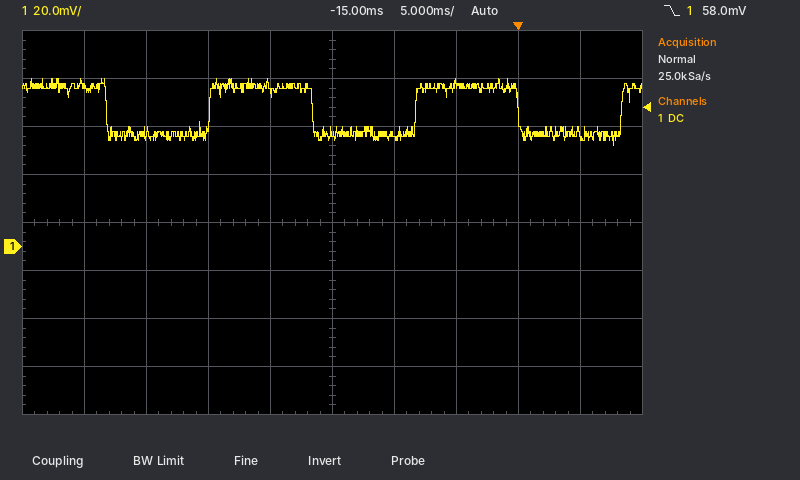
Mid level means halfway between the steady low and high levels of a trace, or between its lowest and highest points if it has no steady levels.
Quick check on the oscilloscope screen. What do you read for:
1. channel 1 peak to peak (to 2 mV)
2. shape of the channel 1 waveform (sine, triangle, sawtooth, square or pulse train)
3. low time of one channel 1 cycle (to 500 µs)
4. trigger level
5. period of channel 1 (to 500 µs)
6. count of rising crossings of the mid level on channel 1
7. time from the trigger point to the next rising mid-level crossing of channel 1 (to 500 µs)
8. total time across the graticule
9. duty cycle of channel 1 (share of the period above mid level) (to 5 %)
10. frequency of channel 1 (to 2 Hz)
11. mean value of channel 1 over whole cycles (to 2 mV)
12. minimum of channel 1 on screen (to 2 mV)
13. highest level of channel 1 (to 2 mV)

28 mV
square
8.5 ms
58.0 mV
16.5 ms
3
8.5 ms
50 ms
50 %
60 Hz
56 mV
42 mV
70 mV
